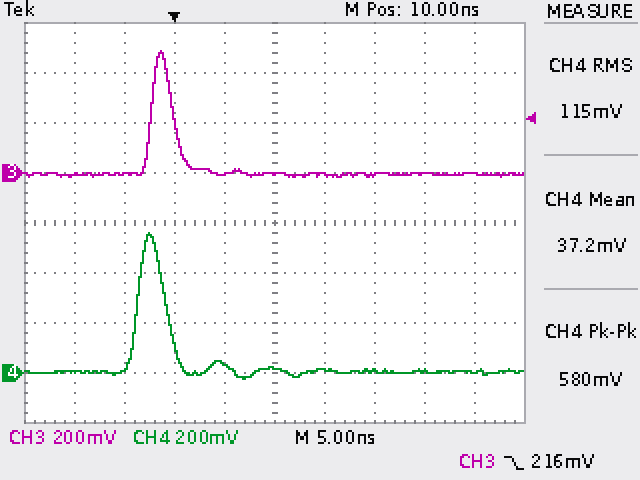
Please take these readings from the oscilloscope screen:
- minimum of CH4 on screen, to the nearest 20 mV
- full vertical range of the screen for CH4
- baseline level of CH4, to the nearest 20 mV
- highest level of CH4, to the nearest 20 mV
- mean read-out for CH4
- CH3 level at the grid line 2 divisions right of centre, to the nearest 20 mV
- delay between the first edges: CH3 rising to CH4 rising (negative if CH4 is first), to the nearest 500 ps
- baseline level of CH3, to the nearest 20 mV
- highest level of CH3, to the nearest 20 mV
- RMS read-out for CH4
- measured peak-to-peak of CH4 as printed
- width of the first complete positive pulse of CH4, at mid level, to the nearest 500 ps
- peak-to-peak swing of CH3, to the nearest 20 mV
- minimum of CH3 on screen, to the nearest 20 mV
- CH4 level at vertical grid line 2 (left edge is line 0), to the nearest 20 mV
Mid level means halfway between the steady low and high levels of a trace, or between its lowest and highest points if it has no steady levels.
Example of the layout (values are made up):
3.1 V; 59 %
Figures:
-20 mV; 1.6 V; 0 mV; 560 mV; 37.2 mV; 0 mV; -1.5 ns; 0 mV; 480 mV; 115 mV; 580 mV; 3.0 ns; 500 mV; -20 mV; 20 mV
